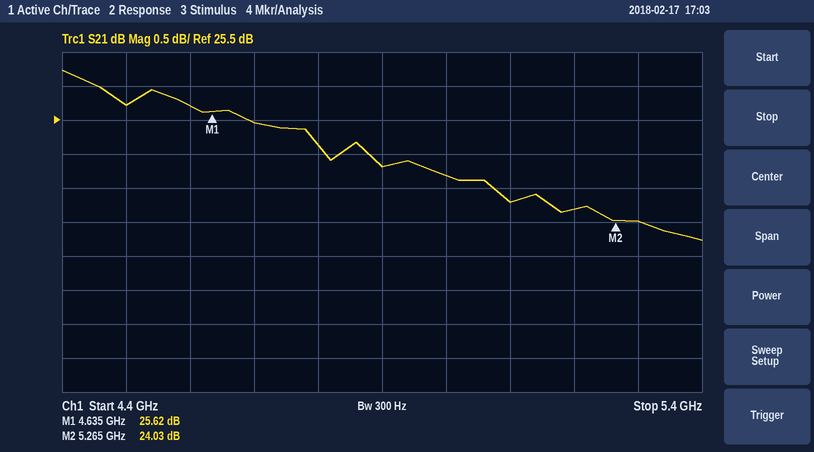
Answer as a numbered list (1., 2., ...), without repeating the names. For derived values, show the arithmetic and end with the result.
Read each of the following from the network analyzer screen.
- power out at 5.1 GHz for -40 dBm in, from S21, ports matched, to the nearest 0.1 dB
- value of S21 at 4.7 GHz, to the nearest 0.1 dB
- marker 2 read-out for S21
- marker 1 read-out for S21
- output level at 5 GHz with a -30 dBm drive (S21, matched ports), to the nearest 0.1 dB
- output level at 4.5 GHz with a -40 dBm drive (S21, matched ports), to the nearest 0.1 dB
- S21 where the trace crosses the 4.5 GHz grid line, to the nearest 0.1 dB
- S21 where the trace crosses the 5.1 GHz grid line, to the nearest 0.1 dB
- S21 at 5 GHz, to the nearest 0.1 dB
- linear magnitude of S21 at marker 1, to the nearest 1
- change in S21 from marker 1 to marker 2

1. -40 dBm + (24.3 dB) = -15.7 dBm
2. 25.5 dB
3. 24.03 dB
4. 25.62 dB
5. -30 dBm + (24.7 dB) = -5.3 dBm
6. -40 dBm + (25.7 dB) = -14.3 dBm
7. 25.7 dB
8. 24.3 dB
9. 24.7 dB
10. 10^(25.62/20) ≈ 19
11. 24.03 − (25.62) = -1.59 dB
